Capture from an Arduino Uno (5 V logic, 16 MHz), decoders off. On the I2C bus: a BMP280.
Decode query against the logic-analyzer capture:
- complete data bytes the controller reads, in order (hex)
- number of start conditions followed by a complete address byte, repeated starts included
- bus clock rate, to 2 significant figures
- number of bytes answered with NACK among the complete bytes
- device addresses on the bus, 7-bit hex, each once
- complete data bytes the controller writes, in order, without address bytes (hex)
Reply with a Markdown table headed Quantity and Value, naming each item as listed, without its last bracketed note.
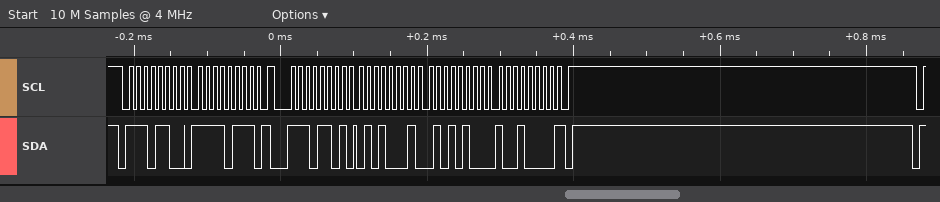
| Quantity | Value |
|---|---|
| complete data bytes the controller reads, in order | 51 54 90 |
| number of start conditions followed by a complete address byte, repeated starts included | 2 |
| bus clock rate, to 2 significant figures | 100 kHz |
| number of bytes answered with NACK among the complete bytes | 1 |
| device addresses on the bus, 7-bit hex, each once | 0x76 |
| complete data bytes the controller writes, in order, without address bytes | F7 |
